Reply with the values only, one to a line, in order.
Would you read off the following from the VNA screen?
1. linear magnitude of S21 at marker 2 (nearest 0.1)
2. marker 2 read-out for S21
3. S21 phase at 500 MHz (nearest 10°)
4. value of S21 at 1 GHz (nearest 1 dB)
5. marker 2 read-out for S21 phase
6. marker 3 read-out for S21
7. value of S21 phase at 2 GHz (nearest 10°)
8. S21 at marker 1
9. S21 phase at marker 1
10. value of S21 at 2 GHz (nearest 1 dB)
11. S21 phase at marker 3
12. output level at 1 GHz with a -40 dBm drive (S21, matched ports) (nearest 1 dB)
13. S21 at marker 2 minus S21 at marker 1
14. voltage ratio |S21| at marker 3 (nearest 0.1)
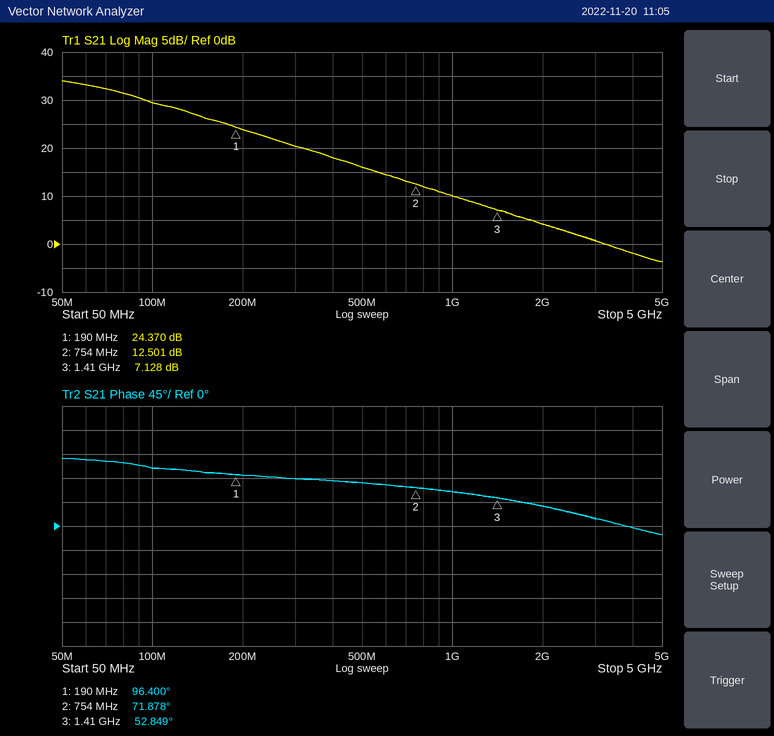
4.2
12.501 dB
80°
10 dB
71.878°
7.128 dB
40°
24.370 dB
96.400°
4 dB
52.849°
-30 dBm
-11.869 dB
2.3
